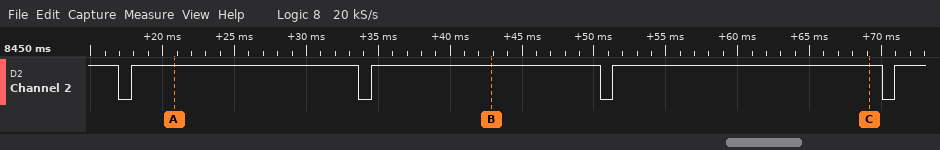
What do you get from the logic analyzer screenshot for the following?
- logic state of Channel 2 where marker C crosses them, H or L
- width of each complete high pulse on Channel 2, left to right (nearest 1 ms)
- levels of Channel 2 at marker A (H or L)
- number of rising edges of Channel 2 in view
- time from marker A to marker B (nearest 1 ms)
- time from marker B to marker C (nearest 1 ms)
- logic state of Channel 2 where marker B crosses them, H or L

Channel 2=H
16 ms, 16 ms, 19 ms
Channel 2=H
4
22 ms
26 ms
Channel 2=H
